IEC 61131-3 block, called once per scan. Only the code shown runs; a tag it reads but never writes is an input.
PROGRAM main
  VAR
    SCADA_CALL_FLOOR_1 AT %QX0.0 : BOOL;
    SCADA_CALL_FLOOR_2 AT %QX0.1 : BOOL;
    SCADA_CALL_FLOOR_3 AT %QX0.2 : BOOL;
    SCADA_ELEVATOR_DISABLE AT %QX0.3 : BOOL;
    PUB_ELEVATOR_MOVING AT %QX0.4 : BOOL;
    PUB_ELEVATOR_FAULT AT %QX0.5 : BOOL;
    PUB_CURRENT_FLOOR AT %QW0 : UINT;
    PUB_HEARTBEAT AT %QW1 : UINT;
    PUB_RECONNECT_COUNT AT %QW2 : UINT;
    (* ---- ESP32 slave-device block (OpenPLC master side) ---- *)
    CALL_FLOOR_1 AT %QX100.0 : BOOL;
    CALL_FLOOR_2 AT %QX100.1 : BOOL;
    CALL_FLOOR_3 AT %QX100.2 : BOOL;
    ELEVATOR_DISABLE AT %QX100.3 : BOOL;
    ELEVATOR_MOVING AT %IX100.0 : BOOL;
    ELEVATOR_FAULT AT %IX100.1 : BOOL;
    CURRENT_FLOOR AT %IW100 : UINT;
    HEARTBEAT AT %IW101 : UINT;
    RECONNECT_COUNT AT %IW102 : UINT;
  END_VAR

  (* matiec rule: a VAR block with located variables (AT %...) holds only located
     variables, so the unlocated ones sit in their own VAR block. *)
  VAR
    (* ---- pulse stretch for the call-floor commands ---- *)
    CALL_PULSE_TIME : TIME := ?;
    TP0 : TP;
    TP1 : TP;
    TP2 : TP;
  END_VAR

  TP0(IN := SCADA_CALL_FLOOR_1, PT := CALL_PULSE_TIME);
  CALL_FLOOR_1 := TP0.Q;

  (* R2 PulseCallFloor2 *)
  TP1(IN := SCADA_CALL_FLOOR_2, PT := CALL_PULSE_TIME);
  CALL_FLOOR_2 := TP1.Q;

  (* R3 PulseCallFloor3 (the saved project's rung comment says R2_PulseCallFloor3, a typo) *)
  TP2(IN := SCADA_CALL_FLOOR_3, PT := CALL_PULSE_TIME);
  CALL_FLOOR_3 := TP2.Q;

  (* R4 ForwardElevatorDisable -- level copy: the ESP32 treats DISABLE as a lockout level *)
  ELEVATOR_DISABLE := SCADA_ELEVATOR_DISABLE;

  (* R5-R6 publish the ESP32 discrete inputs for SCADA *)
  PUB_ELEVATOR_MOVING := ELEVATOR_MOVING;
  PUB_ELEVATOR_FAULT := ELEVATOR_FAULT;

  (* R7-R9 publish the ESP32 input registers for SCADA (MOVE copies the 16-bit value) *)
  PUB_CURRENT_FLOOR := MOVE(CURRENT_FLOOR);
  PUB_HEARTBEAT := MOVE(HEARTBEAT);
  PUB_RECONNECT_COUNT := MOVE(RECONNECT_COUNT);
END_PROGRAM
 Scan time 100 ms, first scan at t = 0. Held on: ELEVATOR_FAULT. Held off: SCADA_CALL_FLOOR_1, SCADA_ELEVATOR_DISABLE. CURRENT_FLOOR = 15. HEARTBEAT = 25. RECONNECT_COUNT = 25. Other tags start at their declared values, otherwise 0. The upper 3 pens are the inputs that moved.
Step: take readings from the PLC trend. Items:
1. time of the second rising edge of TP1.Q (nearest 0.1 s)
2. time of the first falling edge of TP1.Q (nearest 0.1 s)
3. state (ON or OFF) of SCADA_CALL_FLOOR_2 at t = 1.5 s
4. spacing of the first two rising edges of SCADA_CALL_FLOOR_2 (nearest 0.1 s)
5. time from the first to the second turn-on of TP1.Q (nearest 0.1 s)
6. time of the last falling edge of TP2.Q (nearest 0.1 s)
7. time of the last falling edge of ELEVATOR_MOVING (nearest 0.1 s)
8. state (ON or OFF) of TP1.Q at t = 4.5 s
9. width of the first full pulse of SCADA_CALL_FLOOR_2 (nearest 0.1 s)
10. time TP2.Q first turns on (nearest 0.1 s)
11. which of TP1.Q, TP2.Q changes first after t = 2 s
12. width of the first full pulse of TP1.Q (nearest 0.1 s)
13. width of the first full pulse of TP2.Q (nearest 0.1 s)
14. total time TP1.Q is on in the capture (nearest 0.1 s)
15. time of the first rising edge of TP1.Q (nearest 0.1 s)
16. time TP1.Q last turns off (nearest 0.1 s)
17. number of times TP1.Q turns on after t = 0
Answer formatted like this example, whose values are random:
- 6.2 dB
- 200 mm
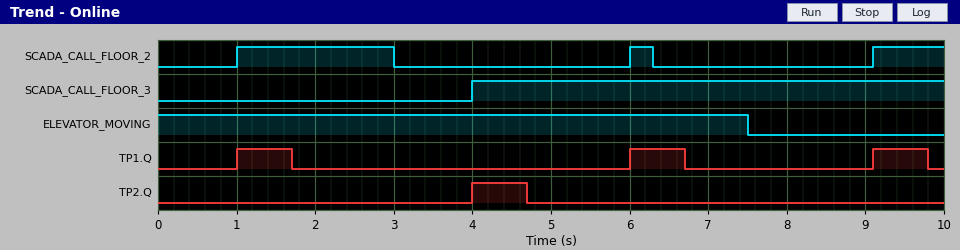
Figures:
- 6.0 s
- 1.7 s
- ON
- 5.0 s
- 5.0 s
- 4.7 s
- 7.5 s
- OFF
- 2.0 s
- 4.0 s
- TP2.Q
- 0.7 s
- 0.7 s
- 2.1 s
- 1.0 s
- 9.8 s
- 3
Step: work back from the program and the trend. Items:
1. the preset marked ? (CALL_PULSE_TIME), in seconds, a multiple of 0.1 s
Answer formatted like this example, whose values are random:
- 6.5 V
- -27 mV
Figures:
- 0.7 s
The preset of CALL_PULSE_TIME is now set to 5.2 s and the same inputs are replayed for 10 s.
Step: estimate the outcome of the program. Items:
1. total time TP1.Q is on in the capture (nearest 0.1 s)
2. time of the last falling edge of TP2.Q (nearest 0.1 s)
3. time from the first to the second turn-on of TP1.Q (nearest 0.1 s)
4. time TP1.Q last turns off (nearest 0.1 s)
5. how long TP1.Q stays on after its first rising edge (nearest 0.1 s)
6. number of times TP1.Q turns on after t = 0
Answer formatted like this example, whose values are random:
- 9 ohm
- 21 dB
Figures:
- 6.1 s
- 9.2 s
- 8.1 s
- 6.2 s
- 5.2 s
- 2
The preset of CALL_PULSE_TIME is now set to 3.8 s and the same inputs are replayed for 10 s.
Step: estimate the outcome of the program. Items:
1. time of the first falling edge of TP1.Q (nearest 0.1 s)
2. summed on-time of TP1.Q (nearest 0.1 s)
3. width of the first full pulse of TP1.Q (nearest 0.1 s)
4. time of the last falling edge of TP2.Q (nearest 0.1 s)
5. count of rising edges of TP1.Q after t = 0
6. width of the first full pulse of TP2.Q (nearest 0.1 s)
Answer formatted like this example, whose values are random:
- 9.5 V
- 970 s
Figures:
- 4.8 s
- 7.6 s
- 3.8 s
- 7.8 s
- 2
- 3.8 s
